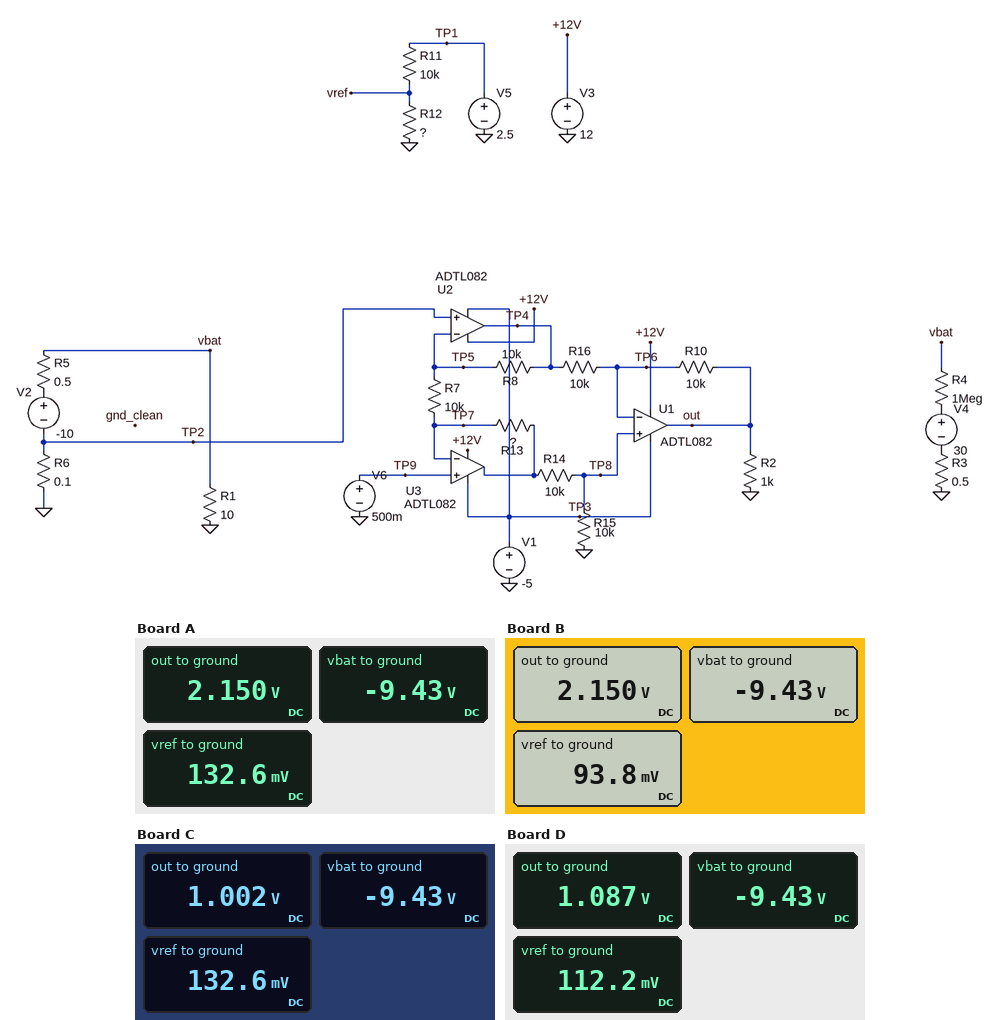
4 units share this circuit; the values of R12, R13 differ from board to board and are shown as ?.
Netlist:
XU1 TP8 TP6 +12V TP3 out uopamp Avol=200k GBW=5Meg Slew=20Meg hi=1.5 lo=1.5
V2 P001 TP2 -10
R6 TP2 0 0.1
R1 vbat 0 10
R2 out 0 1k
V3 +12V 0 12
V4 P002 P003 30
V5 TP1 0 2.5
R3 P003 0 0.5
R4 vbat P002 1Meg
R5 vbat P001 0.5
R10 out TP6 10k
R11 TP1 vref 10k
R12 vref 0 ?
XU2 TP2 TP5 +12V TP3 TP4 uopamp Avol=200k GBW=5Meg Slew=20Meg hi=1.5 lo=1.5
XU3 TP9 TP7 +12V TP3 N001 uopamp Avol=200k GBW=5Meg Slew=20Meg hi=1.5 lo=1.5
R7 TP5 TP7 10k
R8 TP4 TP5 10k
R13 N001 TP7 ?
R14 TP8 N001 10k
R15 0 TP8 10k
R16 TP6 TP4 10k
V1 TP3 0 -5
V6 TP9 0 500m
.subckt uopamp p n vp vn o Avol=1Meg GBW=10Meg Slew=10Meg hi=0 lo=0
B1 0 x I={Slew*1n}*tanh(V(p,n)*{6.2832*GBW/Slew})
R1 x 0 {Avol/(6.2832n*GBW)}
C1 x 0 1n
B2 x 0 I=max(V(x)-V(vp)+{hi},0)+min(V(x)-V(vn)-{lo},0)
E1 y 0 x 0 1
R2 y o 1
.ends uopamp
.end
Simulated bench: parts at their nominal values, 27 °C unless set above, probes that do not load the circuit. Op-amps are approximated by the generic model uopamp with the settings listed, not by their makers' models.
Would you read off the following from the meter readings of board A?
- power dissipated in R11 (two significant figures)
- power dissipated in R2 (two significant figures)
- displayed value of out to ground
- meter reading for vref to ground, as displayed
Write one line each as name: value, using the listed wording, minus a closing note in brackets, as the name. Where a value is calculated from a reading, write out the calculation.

power dissipated in R11: (2.5 V - 132.6 mV)^2 / 10 kΩ = 560 µW
power dissipated in R2: (2.15 V)^2 / 1 kΩ = 4.6 mW
displayed value of out to ground: 2.150 V
meter reading for vref to ground, as displayed: 132.6 mV
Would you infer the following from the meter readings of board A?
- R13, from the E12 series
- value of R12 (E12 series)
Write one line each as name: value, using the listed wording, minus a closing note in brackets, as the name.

R13, from the E12 series: 33 kΩ
value of R12: 560 Ω
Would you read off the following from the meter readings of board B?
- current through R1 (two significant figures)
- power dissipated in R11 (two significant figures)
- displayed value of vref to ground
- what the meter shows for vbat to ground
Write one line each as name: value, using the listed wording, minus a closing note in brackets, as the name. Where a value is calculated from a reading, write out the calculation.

current through R1: (0 V - (-9.43 V)) / 10 Ω = 940 mA
power dissipated in R11: (2.5 V - 93.8 mV)^2 / 10 kΩ = 580 µW
displayed value of vref to ground: 93.8 mV
what the meter shows for vbat to ground: -9.43 V
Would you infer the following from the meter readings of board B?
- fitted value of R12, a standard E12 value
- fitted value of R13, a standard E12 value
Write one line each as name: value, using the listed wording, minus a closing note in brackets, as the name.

fitted value of R12, a standard E12 value: 390 Ω
fitted value of R13, a standard E12 value: 33 kΩ
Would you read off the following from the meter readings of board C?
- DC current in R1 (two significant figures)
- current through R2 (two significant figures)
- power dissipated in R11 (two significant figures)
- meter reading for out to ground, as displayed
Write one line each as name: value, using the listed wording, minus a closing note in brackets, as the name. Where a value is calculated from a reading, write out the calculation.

DC current in R1: (0 V - (-9.43 V)) / 10 Ω = 940 mA
current through R2: (1.002 V) / 1 kΩ = 1.0 mA
power dissipated in R11: (2.5 V - 132.6 mV)^2 / 10 kΩ = 560 µW
meter reading for out to ground, as displayed: 1.002 V
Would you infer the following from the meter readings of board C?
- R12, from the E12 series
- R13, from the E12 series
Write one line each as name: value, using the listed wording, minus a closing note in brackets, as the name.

R12, from the E12 series: 560 Ω
R13, from the E12 series: 4.7 kΩ
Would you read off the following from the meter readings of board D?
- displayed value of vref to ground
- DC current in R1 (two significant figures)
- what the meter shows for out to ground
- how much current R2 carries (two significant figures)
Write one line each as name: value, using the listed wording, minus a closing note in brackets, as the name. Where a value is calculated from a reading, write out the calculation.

displayed value of vref to ground: 112.2 mV
DC current in R1: (0 V - (-9.43 V)) / 10 Ω = 940 mA
what the meter shows for out to ground: 1.087 V
how much current R2 carries: (1.087 V) / 1 kΩ = 1.1 mA
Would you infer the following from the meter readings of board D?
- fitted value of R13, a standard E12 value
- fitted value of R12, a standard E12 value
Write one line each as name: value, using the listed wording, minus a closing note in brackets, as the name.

fitted value of R13, a standard E12 value: 6.8 kΩ
fitted value of R12, a standard E12 value: 470 Ω
